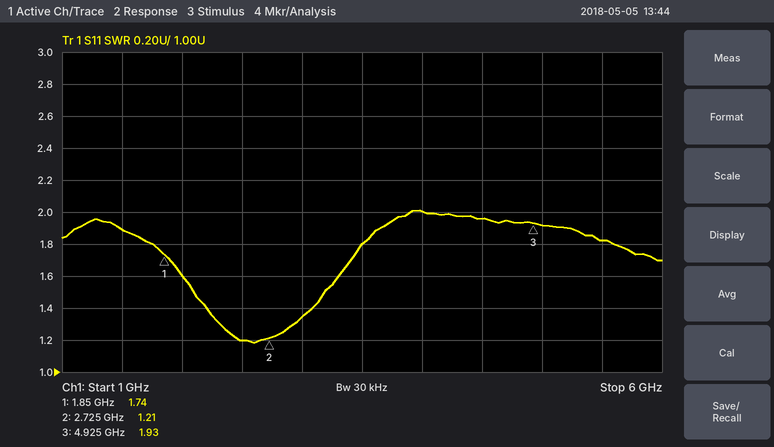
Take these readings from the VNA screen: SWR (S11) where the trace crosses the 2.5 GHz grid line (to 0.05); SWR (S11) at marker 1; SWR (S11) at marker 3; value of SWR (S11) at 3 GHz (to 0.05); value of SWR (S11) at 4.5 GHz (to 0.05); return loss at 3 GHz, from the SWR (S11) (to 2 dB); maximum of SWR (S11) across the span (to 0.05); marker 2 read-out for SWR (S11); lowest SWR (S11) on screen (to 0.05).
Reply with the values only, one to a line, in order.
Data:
1.20
1.74
1.93
1.35
1.95
16 dB
2.00
1.21
1.20
